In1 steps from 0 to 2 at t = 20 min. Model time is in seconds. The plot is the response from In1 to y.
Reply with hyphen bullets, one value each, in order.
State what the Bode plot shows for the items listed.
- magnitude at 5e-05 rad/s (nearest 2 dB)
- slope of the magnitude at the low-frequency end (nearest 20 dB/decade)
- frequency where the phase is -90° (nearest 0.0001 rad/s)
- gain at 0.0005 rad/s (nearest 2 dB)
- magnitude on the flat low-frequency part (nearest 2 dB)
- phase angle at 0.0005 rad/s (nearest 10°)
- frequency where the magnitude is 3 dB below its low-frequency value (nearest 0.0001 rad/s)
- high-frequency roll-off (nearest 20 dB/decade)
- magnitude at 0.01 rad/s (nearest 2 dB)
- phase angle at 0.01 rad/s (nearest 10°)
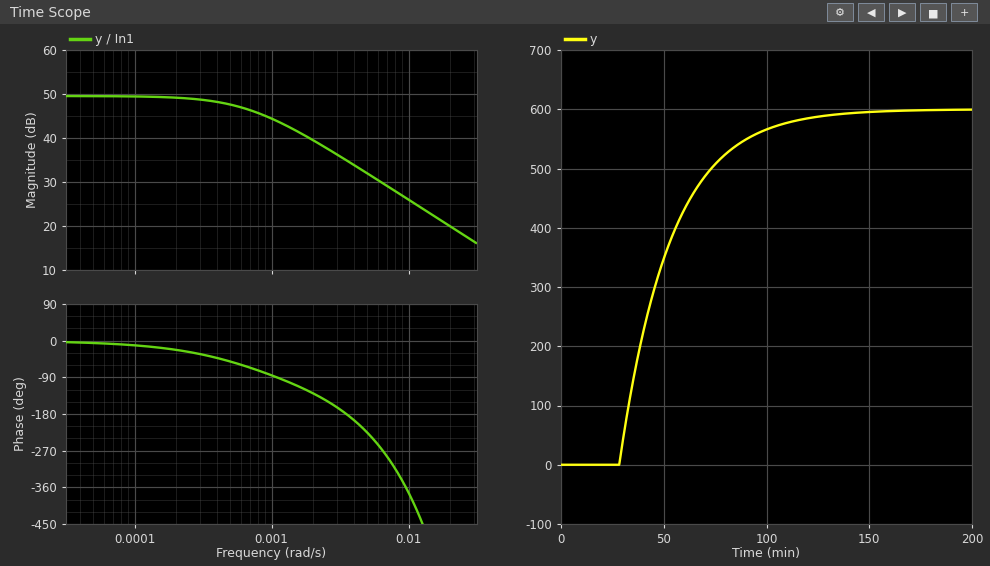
- 50 dB
- 0 dB/decade
- 0.0011 rad/s
- 48 dB
- 50 dB
- -50°
- 0.0007 rad/s
- -20 dB/decade
- 26 dB
- -370°
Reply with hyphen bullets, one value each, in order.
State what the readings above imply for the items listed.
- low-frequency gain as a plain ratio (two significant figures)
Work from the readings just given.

- 320
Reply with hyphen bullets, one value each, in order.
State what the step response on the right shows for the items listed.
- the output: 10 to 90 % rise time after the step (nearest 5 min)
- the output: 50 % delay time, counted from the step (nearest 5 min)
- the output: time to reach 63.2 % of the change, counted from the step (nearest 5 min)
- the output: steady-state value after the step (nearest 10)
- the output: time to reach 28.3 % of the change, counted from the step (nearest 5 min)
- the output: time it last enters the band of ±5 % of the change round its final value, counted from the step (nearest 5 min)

- 55 min
- 25 min
- 35 min
- 600
- 15 min
- 85 min
